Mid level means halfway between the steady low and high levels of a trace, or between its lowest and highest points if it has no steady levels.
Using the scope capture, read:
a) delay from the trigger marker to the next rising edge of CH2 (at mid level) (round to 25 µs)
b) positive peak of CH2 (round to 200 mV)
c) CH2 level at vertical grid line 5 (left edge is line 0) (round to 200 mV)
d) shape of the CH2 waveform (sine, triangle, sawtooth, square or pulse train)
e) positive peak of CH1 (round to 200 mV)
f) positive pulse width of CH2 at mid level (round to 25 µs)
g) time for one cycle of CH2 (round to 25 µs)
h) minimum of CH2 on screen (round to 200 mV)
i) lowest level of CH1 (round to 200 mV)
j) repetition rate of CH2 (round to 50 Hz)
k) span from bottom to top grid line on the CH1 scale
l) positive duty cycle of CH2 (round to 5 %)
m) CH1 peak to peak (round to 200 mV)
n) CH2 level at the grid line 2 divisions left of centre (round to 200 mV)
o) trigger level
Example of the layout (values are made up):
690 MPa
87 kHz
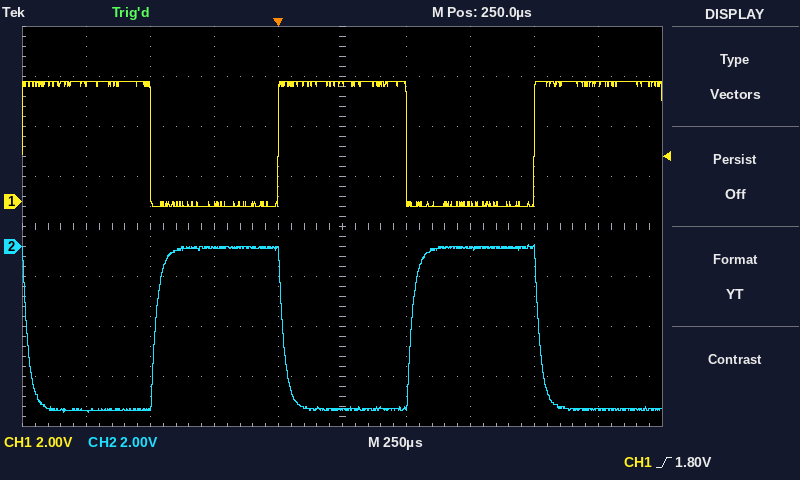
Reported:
525 µs
0.0 V
-6.6 V
square
4.8 V
500 µs
1.000 ms
-6.6 V
-200 mV
1.00 kHz
16 V
50 %
5.0 V
0.0 V
1.80 V
